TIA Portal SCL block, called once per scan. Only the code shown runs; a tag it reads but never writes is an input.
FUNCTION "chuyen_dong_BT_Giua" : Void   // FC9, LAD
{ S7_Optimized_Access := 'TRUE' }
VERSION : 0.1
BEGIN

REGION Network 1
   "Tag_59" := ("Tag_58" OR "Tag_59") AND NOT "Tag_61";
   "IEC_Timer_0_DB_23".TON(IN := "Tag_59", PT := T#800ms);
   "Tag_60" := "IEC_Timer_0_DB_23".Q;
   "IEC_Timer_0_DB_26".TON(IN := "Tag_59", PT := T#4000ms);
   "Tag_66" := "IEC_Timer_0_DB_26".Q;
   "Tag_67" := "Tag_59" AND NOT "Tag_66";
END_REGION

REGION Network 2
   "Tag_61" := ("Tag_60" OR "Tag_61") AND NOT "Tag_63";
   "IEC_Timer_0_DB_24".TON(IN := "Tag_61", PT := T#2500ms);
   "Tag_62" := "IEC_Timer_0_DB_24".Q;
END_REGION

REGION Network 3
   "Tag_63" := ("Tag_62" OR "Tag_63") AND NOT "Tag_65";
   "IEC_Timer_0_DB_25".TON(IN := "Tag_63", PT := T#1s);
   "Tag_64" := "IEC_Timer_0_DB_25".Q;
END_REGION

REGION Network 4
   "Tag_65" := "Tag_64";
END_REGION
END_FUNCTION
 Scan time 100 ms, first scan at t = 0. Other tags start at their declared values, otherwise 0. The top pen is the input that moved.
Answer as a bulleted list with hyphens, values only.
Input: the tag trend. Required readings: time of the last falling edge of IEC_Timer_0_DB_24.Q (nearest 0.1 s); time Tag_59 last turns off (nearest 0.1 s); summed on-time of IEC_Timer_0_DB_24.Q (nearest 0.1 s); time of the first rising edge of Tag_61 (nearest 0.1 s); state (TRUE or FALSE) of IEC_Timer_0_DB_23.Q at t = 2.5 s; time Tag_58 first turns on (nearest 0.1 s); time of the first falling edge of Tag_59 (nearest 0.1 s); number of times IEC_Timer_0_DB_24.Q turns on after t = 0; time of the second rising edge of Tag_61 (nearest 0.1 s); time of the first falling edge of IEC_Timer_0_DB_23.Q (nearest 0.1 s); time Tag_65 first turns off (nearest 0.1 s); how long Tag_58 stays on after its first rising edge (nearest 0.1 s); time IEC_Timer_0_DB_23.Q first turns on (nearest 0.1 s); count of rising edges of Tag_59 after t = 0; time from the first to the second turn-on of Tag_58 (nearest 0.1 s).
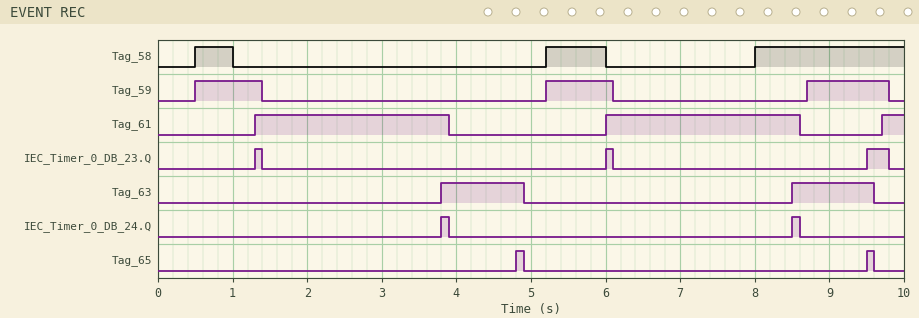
- 8.6 s
- 9.8 s
- 0.2 s
- 1.3 s
- FALSE
- 0.5 s
- 1.4 s
- 2
- 6.0 s
- 1.4 s
- 4.9 s
- 0.5 s
- 1.3 s
- 3
- 4.7 s
